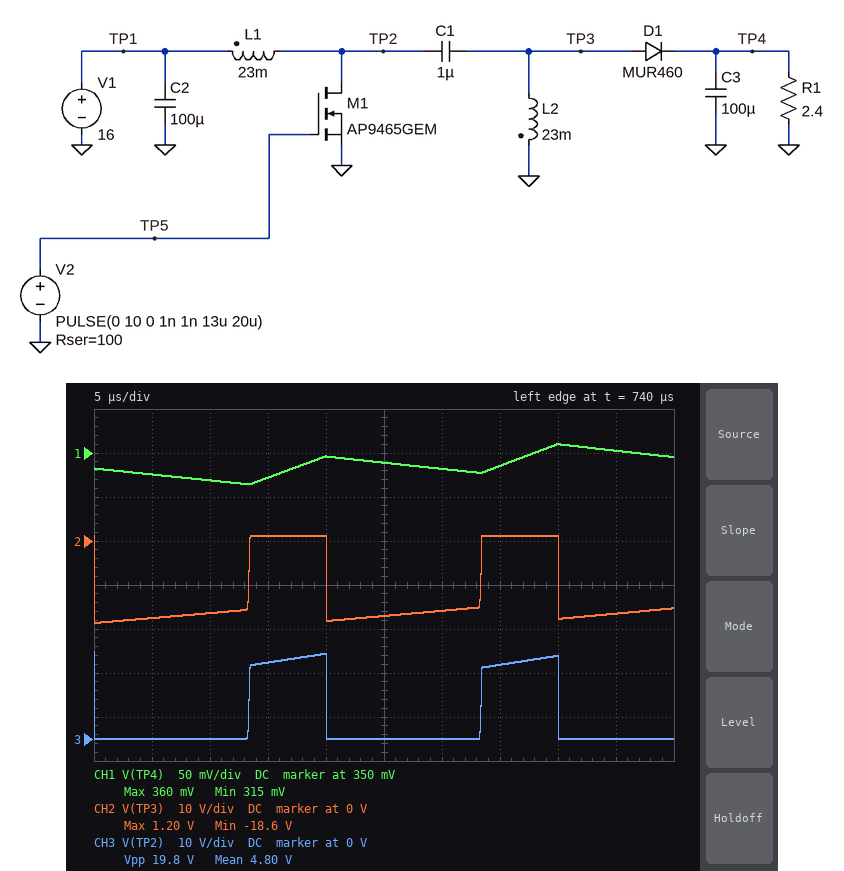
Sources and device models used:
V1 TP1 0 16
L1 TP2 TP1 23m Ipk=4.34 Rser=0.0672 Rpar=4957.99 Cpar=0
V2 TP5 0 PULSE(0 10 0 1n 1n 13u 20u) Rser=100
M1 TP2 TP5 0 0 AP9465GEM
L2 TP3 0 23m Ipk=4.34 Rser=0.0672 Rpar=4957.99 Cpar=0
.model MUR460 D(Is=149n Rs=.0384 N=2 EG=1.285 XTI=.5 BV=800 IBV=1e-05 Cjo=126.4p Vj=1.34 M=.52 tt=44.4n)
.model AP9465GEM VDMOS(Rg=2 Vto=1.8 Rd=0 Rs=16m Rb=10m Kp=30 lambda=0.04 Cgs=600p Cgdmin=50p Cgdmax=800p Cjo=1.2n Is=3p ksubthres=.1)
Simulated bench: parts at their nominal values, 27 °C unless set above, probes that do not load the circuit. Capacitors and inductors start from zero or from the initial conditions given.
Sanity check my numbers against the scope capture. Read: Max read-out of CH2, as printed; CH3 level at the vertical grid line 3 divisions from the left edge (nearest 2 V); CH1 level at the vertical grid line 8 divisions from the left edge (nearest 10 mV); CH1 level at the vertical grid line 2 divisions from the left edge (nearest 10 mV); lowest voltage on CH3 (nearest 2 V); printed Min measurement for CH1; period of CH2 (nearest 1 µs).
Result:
1.20 V
18 V
360 mV
320 mV
0 V
315 mV
20 µs
